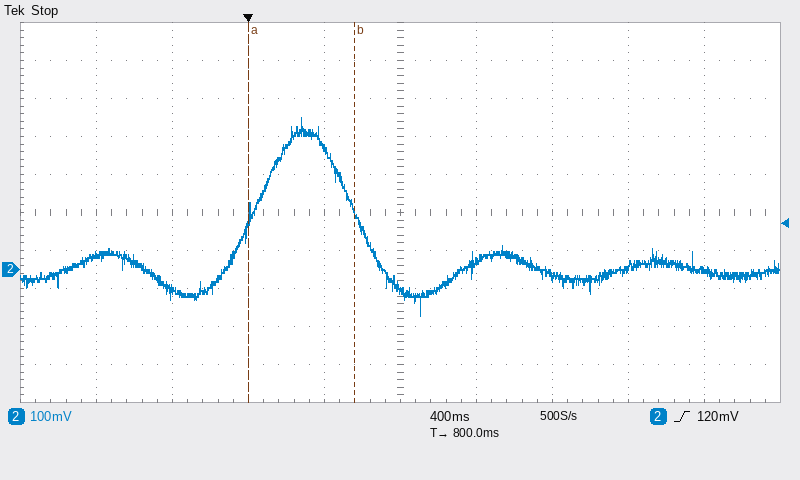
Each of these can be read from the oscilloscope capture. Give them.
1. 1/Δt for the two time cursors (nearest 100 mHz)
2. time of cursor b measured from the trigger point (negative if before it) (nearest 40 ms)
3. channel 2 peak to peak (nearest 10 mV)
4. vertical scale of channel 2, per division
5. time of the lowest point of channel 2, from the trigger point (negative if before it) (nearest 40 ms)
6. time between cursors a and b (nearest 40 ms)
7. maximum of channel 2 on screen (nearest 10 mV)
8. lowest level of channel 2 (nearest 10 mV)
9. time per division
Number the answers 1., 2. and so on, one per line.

1. 1.8 Hz
2. +560 ms
3. 520 mV
4. 100 mV
5. +920 ms
6. 560 ms
7. 400 mV
8. -120 mV
9. 400 ms
